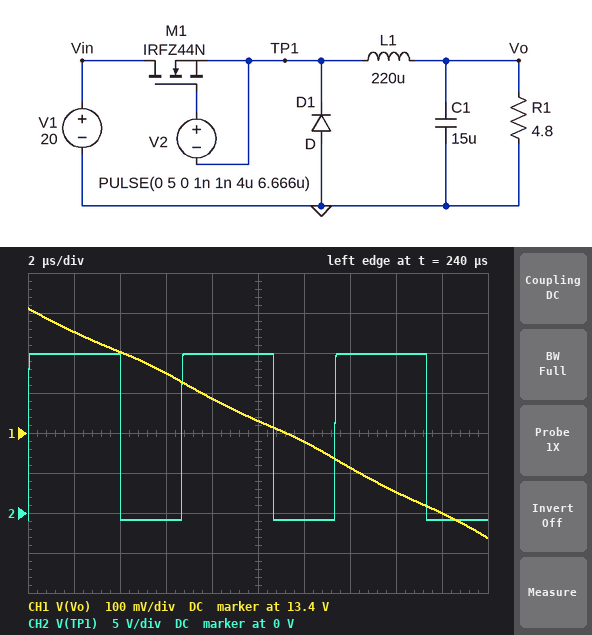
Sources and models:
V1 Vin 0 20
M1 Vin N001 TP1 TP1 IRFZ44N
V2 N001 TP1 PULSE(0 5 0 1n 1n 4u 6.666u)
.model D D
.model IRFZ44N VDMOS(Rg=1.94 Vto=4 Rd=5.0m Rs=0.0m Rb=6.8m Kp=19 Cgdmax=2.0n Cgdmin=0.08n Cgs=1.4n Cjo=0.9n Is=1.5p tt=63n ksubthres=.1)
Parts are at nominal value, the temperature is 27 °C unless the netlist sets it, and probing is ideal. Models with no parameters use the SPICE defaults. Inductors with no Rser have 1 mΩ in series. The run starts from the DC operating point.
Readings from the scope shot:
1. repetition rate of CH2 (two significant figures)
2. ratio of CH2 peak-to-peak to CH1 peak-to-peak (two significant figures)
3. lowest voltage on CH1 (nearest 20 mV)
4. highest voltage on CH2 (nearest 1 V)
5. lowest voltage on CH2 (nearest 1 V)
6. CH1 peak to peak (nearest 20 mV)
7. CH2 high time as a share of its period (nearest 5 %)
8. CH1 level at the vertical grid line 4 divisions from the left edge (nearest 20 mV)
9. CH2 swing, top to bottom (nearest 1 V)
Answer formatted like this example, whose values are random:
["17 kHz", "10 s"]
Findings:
["150 kHz", "36", "13.14 V", "20 V", "-1 V", "580 mV", "60 %", "13.48 V", "21 V"]
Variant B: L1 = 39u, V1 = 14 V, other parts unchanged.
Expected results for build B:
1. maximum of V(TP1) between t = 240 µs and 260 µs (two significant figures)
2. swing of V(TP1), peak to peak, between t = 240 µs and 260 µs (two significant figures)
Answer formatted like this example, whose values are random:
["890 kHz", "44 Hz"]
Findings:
["14 V", "15 V"]
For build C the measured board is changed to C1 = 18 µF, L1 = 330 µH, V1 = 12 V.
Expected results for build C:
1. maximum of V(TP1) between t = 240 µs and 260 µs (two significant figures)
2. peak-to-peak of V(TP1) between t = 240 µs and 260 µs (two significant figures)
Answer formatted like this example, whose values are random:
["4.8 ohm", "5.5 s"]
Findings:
["12 V", "13 V"]
